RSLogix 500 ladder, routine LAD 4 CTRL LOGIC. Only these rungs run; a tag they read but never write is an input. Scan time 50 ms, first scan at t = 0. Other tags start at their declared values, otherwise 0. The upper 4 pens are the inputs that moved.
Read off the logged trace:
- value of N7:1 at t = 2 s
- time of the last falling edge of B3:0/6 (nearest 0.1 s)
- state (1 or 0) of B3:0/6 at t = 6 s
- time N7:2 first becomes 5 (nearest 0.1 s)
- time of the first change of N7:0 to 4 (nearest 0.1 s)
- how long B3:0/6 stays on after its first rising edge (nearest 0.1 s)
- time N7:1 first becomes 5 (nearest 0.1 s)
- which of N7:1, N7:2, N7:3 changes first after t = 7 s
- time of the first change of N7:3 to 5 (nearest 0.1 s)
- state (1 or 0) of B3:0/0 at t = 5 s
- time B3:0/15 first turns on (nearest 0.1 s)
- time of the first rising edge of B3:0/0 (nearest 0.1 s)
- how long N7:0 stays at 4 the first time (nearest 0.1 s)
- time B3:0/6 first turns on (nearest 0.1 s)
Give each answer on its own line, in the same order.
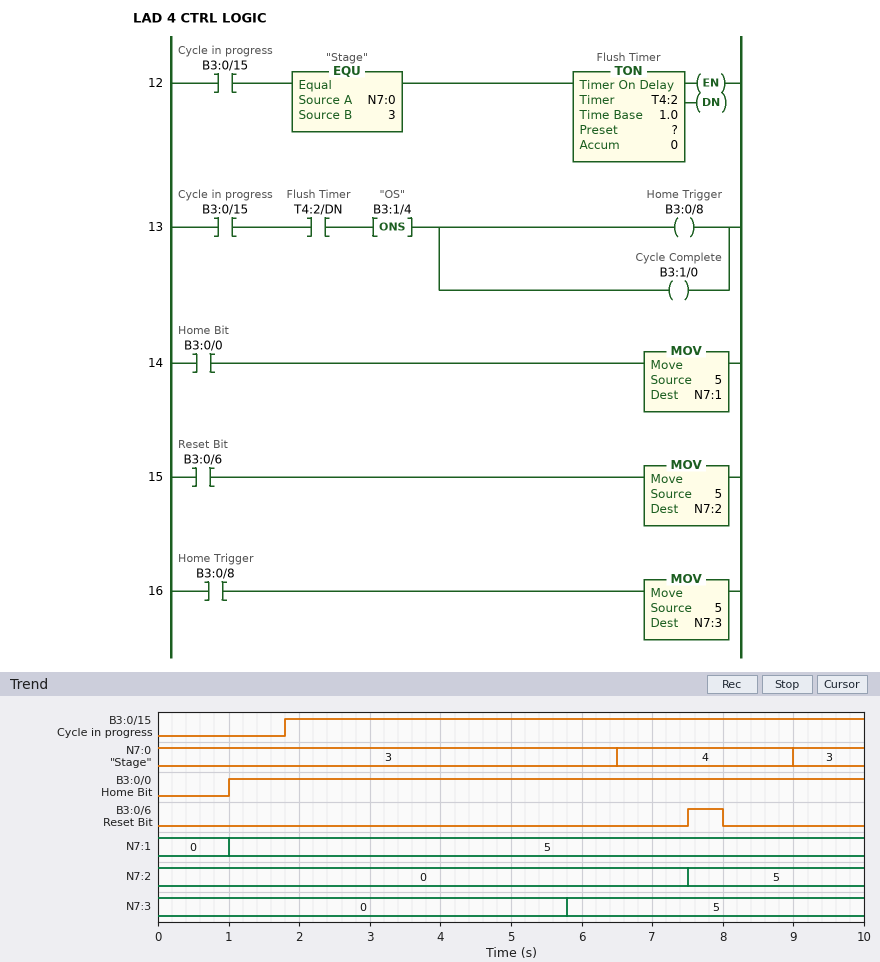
5
8.0 s
0
7.5 s
6.5 s
0.5 s
1.0 s
N7:2
5.8 s
1
1.8 s
1.0 s
2.5 s
7.5 s
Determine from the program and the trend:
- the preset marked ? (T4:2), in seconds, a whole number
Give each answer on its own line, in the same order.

4 s
